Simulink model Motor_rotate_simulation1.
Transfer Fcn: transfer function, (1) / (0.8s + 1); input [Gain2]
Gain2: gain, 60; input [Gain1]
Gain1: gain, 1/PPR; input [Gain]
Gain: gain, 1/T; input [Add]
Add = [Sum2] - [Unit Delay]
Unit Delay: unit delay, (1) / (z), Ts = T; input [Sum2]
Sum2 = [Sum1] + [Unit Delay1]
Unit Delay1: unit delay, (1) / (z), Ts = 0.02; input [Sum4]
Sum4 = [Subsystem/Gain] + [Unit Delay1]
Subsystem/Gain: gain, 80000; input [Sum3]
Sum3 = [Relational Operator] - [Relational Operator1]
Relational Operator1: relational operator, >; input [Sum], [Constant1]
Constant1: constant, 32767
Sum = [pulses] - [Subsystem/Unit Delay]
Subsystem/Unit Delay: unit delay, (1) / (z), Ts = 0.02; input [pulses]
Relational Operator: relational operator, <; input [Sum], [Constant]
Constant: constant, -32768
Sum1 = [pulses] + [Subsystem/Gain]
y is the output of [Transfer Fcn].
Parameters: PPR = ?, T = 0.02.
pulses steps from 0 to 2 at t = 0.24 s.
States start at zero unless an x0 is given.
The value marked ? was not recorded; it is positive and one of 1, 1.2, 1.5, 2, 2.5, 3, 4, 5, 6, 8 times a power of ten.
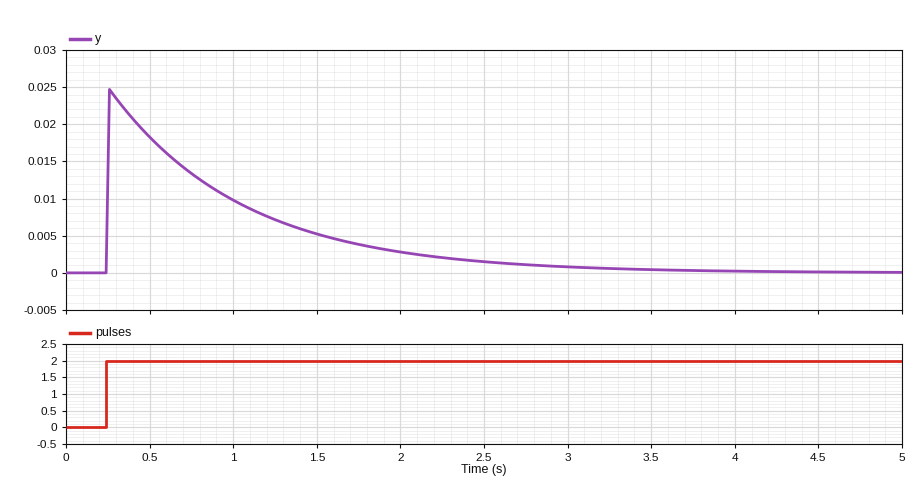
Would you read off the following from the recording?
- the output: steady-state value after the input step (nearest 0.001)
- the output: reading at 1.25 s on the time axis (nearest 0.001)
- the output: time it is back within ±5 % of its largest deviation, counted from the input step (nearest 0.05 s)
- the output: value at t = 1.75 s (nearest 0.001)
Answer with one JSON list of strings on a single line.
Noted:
["0.000", "0.007", "2.40 s", "0.004"]
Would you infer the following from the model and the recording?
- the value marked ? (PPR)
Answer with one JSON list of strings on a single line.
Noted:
["6000"]
